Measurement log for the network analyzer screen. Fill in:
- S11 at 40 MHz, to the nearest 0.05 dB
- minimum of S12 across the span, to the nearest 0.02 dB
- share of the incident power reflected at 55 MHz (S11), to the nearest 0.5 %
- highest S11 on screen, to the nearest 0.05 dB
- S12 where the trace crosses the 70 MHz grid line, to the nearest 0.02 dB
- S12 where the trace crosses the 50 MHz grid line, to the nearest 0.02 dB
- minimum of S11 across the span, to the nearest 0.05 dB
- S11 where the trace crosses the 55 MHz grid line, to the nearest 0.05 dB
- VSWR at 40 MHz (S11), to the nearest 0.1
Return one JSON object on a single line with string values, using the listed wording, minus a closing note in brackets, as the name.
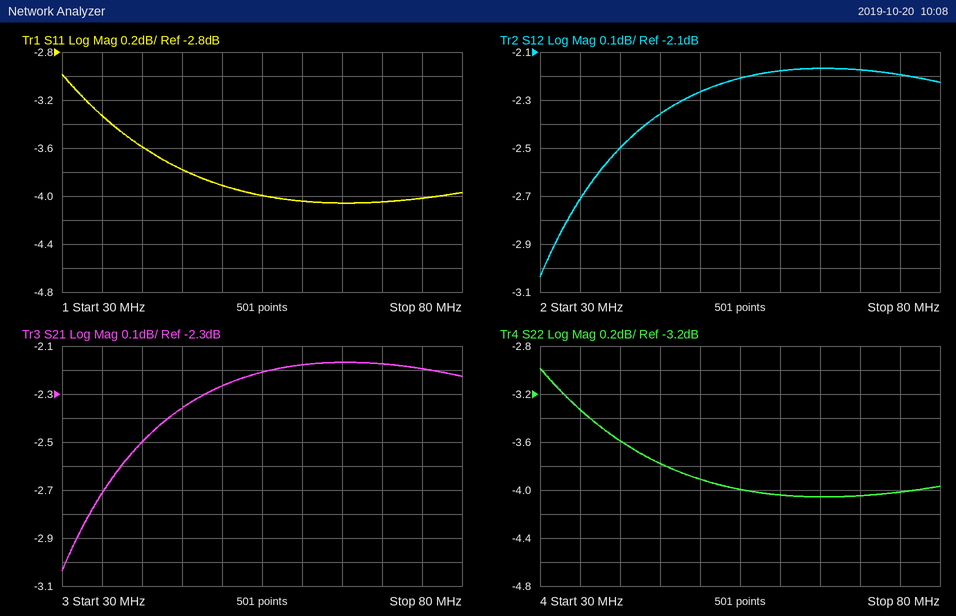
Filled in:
{"S11 at 40 MHz, to the nearest 0.05 dB": "-3.60 dB", "minimum of S12 across the span, to the nearest 0.02 dB": "-3.04 dB", "share of the incident power reflected at 55 MHz (S11), to the nearest 0.5 %": "40.0 %", "highest S11 on screen, to the nearest 0.05 dB": "-3.00 dB", "S12 where the trace crosses the 70 MHz grid line, to the nearest 0.02 dB": "-2.18 dB", "S12 where the trace crosses the 50 MHz grid line, to the nearest 0.02 dB": "-2.26 dB", "minimum of S11 across the span, to the nearest 0.05 dB": "-4.05 dB", "S11 where the trace crosses the 55 MHz grid line, to the nearest 0.05 dB": "-4.00 dB", "VSWR at 40 MHz (S11), to the nearest 0.1": "4.9"}
